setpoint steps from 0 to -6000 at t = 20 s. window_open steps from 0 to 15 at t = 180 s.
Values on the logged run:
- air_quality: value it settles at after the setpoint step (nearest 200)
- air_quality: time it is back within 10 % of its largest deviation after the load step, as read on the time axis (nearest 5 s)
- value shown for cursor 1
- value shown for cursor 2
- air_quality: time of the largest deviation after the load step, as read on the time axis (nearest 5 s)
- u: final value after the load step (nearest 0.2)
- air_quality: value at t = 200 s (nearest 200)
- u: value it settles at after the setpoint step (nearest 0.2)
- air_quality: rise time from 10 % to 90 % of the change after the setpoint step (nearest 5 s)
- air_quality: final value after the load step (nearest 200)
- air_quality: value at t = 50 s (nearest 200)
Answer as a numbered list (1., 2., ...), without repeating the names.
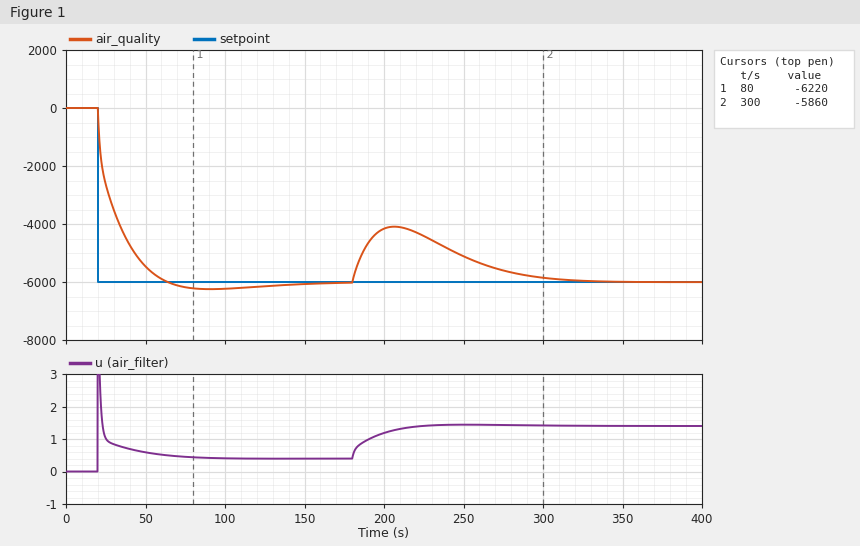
1. -6000
2. 295 s
3. -6220
4. -5860
5. 205 s
6. 1.4
7. -4200
8. 0.4
9. 30 s
10. -6000
11. -5400
